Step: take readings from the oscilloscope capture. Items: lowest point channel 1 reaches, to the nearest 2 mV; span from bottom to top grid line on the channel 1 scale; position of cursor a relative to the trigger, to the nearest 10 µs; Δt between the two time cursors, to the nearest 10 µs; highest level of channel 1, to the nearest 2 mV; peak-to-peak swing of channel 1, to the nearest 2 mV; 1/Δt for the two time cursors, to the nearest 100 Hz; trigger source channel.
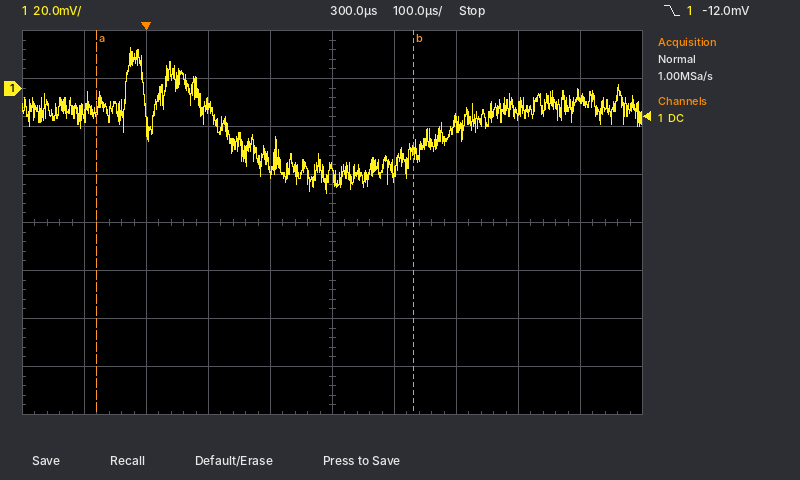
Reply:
-44 mV
160 mV
-80 µs
510 µs
16 mV
60 mV
2.0 kHz
channel 1
